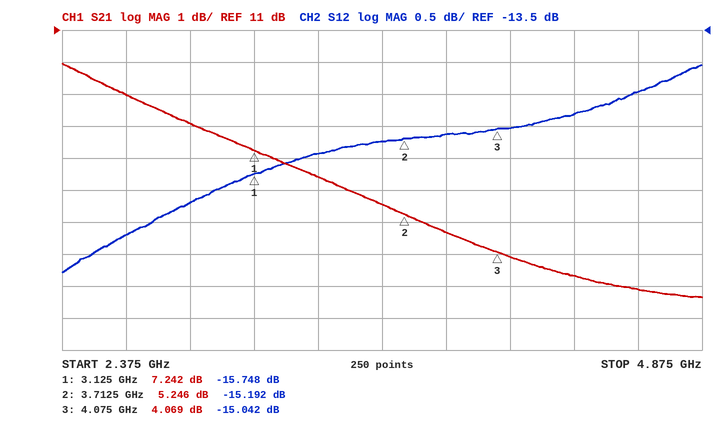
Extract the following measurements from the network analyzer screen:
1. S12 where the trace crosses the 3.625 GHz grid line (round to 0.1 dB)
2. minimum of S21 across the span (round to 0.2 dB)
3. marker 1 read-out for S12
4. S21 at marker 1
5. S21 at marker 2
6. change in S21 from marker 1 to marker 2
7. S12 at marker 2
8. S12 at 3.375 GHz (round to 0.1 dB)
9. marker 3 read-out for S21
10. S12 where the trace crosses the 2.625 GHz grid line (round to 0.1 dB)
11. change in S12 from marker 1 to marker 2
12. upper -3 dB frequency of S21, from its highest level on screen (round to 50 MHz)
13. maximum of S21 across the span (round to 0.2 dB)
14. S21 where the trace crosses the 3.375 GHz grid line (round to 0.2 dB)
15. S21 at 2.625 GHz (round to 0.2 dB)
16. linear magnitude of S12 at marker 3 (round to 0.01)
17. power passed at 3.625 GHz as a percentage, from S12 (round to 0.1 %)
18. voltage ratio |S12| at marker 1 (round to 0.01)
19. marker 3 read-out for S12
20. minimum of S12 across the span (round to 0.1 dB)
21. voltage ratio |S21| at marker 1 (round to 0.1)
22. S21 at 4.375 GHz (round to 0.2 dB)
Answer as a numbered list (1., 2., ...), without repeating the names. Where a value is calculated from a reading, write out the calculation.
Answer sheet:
1. -15.2 dB
2. 2.6 dB
3. -15.748 dB
4. 7.242 dB
5. 5.246 dB
6. 5.246 − (7.242) = -1.996 dB
7. -15.192 dB
8. -15.4 dB
9. 4.069 dB
10. -16.7 dB
11. -15.192 − (-15.748) = 0.556 dB
12. 3.20 GHz
13. 10.0 dB
14. 6.4 dB
15. 9.0 dB
16. 10^(-15.042/20) ≈ 0.18
17. 10^(-15.2/10) ≈ 3.0 %
18. 10^(-15.748/20) ≈ 0.16
19. -15.042 dB
20. -17.3 dB
21. 10^(7.242/20) ≈ 2.3
22. 3.4 dB
